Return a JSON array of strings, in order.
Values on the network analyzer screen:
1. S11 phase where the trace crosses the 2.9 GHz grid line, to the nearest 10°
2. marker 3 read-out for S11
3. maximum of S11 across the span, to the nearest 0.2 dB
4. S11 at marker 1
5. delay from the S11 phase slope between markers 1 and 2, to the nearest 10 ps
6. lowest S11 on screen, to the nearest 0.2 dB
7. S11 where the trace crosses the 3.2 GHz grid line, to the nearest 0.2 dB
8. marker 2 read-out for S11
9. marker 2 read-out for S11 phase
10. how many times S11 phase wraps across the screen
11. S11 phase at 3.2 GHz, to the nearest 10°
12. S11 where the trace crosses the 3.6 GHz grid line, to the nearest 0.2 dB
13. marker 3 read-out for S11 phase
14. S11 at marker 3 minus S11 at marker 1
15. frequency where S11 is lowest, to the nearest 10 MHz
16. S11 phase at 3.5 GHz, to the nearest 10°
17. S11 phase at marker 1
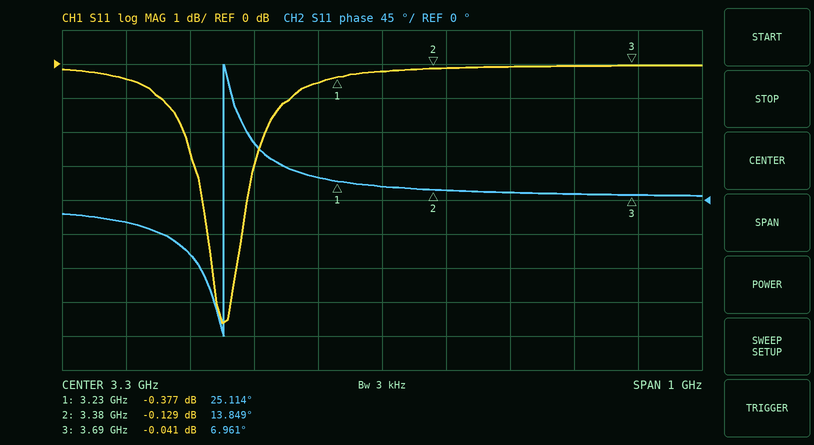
["-30°", "-0.041 dB", "0.0 dB", "-0.377 dB", "210 ps", "-7.6 dB", "-0.6 dB", "-0.129 dB", "13.849°", "1", "30°", "0.0 dB", "6.961°", "0.336 dB", "3.05 GHz", "10°", "25.114°"]
